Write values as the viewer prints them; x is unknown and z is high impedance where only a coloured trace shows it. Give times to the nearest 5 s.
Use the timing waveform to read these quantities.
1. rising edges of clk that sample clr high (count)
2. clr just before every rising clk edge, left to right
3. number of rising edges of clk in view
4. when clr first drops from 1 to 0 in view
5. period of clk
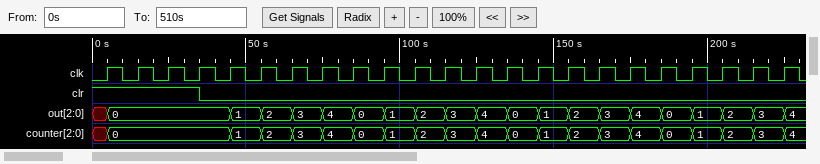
4
1 1 1 1 0 0 0 0 0 0 0 0 0 0 0 0 0 0 0 0 0 0 0
23
35 s
10 s
